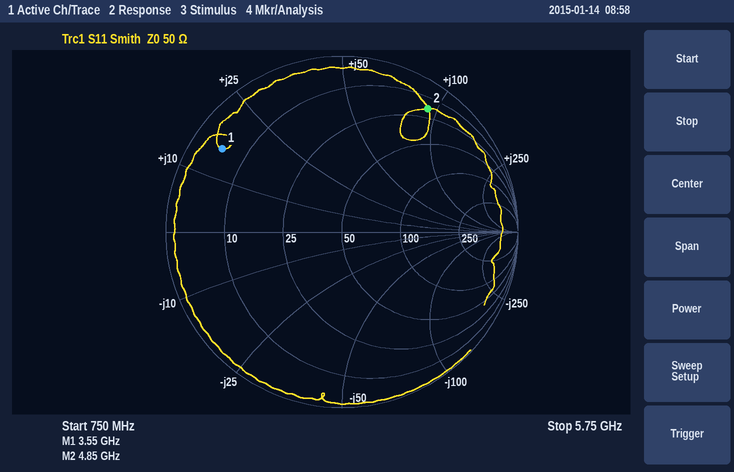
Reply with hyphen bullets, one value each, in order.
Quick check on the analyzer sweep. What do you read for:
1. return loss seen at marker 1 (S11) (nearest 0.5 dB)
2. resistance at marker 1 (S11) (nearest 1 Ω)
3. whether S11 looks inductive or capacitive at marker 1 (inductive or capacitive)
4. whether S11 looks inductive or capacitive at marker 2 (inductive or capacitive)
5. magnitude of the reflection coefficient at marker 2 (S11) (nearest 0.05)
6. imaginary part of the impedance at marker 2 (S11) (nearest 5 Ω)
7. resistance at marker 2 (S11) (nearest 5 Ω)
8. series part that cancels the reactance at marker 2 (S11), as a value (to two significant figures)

- 1.5 dB
- 5 Ω
- inductive
- inductive
- 0.85
- +95 Ω
- 20 Ω
- 350 fF
